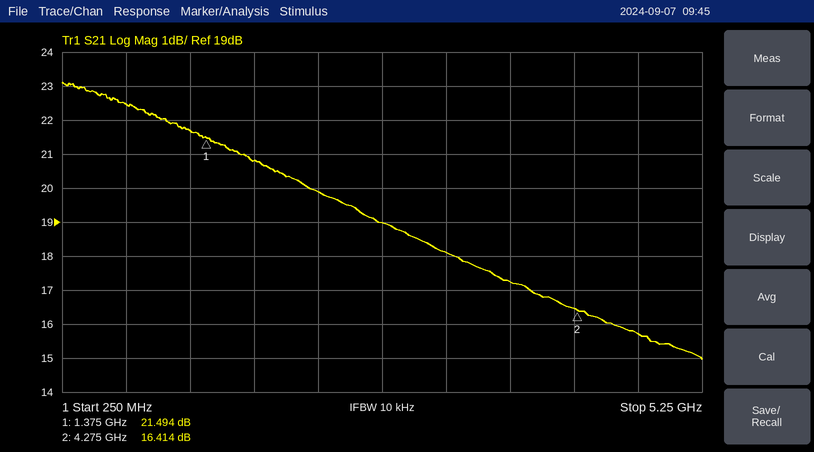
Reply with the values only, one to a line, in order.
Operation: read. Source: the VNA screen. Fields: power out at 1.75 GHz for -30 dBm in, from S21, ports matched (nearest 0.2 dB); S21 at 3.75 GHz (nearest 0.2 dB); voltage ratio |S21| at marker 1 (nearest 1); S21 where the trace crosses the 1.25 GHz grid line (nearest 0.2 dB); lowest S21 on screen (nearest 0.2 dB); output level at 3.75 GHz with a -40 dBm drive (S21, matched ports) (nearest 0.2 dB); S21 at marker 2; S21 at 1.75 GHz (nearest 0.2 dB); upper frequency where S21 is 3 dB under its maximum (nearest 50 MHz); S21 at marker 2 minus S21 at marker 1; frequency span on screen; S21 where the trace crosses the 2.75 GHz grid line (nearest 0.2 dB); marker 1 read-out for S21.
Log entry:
-9.2 dBm
17.2 dB
12
21.6 dB
15.0 dB
-22.8 dBm
16.414 dB
20.8 dB
2.15 GHz
-5.080 dB
5 GHz
19.0 dB
21.494 dB
